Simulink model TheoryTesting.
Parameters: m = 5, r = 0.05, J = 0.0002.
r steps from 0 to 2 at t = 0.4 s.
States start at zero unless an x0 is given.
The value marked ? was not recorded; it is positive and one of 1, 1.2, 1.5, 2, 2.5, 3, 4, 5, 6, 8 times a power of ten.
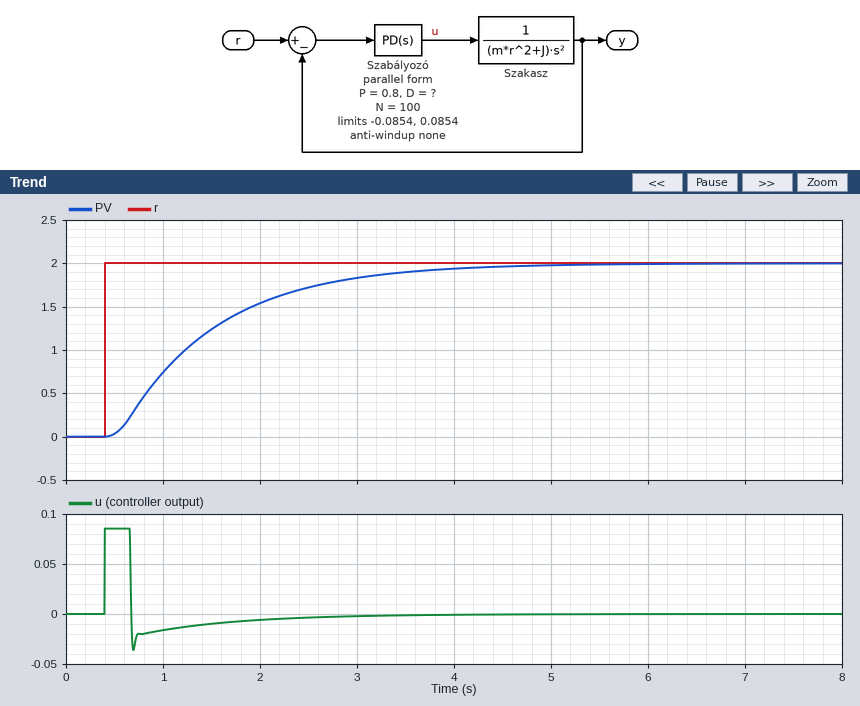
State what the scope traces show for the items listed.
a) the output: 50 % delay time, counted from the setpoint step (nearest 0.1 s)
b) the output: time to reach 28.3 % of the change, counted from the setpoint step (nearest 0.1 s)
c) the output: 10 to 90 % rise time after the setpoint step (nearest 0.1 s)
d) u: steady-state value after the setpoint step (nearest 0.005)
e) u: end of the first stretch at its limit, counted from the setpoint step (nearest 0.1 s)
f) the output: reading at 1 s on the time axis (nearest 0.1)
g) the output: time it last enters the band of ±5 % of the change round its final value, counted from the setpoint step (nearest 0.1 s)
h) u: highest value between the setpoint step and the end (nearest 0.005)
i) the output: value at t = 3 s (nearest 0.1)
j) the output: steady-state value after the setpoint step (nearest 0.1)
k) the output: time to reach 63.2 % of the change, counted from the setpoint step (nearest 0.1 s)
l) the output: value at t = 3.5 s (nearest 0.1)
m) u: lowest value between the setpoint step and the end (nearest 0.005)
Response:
0.8 s
0.5 s
2.2 s
0.000
0.3 s
0.7
3.1 s
0.085
1.8
2.0
1.1 s
1.9
-0.035
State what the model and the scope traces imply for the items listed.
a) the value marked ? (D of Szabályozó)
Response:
0.8
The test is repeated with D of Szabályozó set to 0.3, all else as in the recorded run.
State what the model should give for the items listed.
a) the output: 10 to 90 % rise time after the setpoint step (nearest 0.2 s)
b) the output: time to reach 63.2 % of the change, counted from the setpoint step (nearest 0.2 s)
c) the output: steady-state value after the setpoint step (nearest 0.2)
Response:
0.8 s
0.6 s
2.0
